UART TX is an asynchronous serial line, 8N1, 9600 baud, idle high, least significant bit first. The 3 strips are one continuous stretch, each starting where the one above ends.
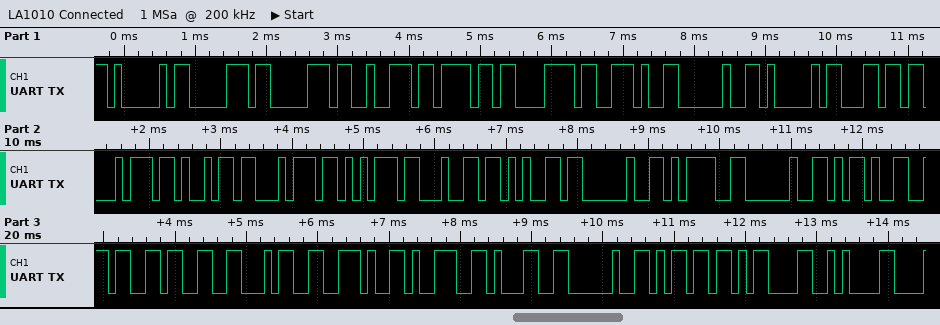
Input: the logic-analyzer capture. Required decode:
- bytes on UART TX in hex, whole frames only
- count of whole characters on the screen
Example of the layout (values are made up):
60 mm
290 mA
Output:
0x41 0x70 0x70 0x72 0x6F 0x78 0x2E 0x20 0x41 0x6C 0x74 0x69 0x74 0x75 0x64 0x65 0x20 0x3D 0x20 0x2D 0x36 0x33 0x34 0x2E 0x39 0x31 0x20 0x6D 0x0D 0x0A
30
